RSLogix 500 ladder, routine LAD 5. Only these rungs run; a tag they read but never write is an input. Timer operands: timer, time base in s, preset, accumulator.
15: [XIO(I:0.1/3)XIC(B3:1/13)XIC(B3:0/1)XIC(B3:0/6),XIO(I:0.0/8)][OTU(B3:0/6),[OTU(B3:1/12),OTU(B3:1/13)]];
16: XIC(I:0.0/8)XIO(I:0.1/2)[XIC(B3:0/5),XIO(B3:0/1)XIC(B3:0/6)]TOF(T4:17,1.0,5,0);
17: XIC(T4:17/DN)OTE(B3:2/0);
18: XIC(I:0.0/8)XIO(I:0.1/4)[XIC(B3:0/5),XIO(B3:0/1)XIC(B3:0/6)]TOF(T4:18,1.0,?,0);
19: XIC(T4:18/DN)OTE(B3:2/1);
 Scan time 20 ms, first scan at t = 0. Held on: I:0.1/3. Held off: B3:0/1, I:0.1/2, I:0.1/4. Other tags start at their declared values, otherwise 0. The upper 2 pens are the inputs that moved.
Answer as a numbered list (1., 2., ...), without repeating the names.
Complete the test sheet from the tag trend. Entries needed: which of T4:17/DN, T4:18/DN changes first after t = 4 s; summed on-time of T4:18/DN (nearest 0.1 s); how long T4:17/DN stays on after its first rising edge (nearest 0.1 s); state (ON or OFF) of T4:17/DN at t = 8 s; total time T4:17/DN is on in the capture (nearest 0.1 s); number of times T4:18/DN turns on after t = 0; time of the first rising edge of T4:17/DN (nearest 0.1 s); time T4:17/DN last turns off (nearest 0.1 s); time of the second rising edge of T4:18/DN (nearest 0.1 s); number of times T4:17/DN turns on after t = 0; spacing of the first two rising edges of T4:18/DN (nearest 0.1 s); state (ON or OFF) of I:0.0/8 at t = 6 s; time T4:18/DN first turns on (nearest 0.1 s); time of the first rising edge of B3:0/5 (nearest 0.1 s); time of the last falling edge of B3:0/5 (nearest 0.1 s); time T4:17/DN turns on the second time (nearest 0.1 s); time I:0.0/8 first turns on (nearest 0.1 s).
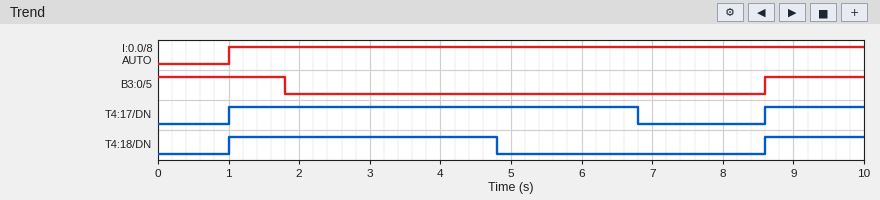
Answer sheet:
1. T4:18/DN
2. 5.2 s
3. 5.8 s
4. OFF
5. 7.2 s
6. 2
7. 1.0 s
8. 6.8 s
9. 8.6 s
10. 2
11. 7.6 s
12. ON
13. 1.0 s
14. 8.6 s
15. 1.8 s
16. 8.6 s
17. 1.0 s
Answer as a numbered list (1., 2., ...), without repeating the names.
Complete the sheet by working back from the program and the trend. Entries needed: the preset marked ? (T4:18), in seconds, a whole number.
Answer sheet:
1. 3 s
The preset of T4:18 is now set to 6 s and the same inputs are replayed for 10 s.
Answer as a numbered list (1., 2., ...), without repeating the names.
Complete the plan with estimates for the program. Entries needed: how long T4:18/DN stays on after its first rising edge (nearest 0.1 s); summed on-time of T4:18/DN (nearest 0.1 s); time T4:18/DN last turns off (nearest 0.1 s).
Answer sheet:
1. 6.8 s
2. 8.2 s
3. 7.8 s
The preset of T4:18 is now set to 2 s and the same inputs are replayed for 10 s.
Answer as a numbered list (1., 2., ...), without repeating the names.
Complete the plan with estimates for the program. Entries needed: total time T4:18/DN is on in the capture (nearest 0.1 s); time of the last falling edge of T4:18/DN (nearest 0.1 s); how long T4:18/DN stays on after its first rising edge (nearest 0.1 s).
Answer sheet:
1. 4.2 s
2. 3.8 s
3. 2.8 s
